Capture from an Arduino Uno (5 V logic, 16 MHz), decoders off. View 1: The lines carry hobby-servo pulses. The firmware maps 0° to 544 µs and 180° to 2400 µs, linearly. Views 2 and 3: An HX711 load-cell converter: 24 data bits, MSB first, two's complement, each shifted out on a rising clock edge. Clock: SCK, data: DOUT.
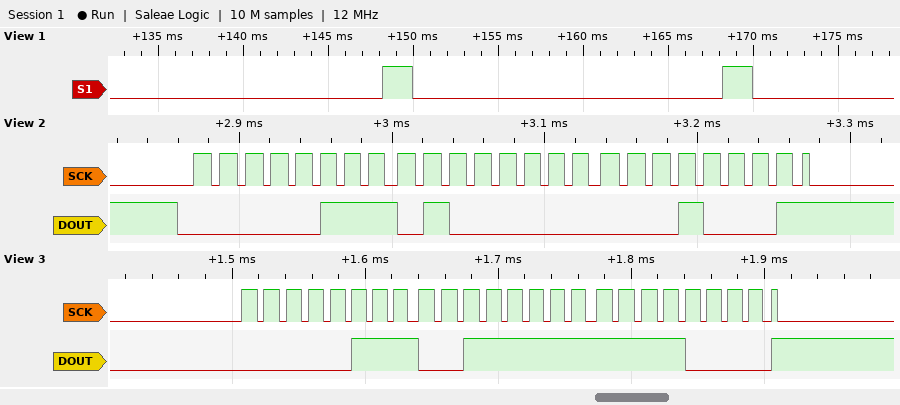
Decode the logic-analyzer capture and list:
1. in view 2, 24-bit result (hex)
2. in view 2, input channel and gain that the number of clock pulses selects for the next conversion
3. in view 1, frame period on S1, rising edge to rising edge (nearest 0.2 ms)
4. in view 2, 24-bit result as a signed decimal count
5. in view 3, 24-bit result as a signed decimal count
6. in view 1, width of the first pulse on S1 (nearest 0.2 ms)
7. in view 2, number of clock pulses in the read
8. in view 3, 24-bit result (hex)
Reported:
0x074011
channel A, gain 128
20.0 ms
475153
475120
1.8 ms
25
0x073FF0
